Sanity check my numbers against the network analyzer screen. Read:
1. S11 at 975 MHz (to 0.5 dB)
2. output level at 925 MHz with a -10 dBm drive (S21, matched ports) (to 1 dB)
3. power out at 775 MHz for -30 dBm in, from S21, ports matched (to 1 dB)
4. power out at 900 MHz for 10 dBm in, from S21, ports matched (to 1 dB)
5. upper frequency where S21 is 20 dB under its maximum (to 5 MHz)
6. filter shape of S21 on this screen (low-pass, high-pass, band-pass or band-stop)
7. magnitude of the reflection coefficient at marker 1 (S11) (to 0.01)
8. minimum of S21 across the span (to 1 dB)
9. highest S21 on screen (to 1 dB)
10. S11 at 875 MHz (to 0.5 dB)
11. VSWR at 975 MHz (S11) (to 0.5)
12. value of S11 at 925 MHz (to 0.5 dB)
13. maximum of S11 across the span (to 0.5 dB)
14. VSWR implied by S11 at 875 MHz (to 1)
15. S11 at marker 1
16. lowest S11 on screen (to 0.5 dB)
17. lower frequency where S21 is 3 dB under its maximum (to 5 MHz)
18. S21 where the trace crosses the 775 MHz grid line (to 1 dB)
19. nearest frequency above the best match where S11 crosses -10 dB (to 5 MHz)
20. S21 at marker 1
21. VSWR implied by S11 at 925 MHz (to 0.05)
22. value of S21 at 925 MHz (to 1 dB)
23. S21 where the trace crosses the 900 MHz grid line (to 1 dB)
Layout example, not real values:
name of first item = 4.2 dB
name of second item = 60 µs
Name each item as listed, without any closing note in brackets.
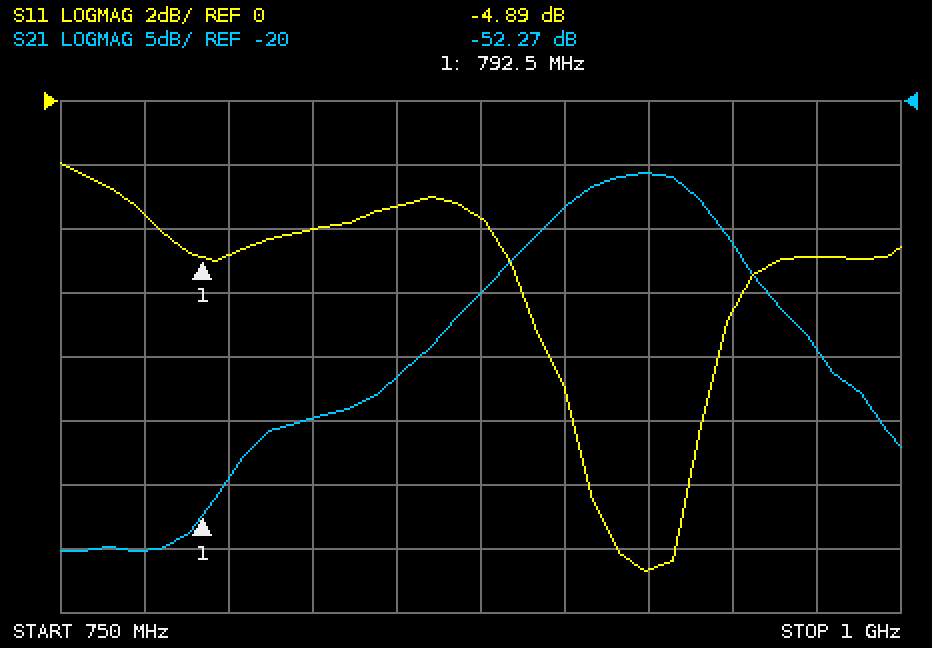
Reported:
S11 at 975 MHz = -5.0 dB
output level at 925 MHz with a -10 dBm drive (S21, matched ports) = -36 dBm
power out at 775 MHz for -30 dBm in, from S21, ports matched = -85 dBm
power out at 900 MHz for 10 dBm in, from S21, ports matched = -18 dBm
upper frequency where S21 is 20 dB under its maximum = 995 MHz
filter shape of S21 on this screen = band-pass
magnitude of the reflection coefficient at marker 1 (S11) = 0.57
minimum of S21 across the span = -55 dB
highest S21 on screen = -26 dB
S11 at 875 MHz = -3.5 dB
VSWR at 975 MHz (S11) = 3.5
value of S11 at 925 MHz = -14.5 dB
maximum of S11 across the span = -2.0 dB
VSWR implied by S11 at 875 MHz = 5
S11 at marker 1 = -4.89 dB
lowest S11 on screen = -14.5 dB
lower frequency where S21 is 3 dB under its maximum = 900 MHz
S21 where the trace crosses the 775 MHz grid line = -55 dB
nearest frequency above the best match where S11 crosses -10 dB = 940 MHz
S21 at marker 1 = -52.27 dB
VSWR implied by S11 at 925 MHz = 1.45
value of S21 at 925 MHz = -26 dB
S21 where the trace crosses the 900 MHz grid line = -28 dB
